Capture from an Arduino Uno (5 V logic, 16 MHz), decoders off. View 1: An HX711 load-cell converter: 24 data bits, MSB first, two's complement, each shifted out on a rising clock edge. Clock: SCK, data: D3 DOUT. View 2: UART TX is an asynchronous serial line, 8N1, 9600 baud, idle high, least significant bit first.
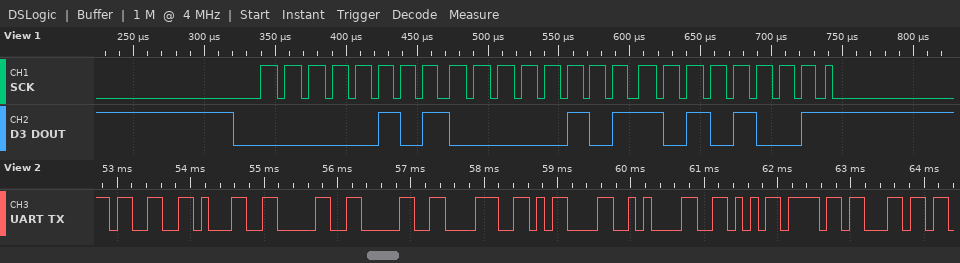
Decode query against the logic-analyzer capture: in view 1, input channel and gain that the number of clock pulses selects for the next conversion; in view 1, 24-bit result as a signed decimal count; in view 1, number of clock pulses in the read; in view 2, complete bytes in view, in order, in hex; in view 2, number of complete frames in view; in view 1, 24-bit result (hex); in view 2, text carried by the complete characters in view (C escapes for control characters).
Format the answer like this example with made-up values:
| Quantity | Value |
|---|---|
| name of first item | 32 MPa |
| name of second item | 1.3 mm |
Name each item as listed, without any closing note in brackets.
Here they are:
| Quantity | Value |
|---|---|
| in view 1, input channel and gain that the number of clock pulses selects for the next conversion | channel A, gain 128 |
| in view 1, 24-bit result as a signed decimal count | 329129 |
| in view 1, number of clock pulses in the read | 25 |
| in view 2, complete bytes in view, in order, in hex | 33 31 30 30 38 0D 0A 56 6F 6C |
| in view 2, number of complete frames in view | 10 |
| in view 1, 24-bit result | 0x0505A9 |
| in view 2, text carried by the complete characters in view | "31008\r\nVol" |
